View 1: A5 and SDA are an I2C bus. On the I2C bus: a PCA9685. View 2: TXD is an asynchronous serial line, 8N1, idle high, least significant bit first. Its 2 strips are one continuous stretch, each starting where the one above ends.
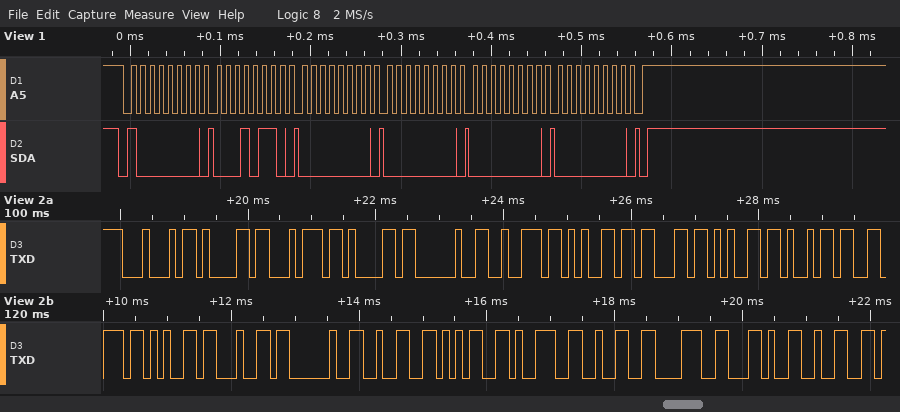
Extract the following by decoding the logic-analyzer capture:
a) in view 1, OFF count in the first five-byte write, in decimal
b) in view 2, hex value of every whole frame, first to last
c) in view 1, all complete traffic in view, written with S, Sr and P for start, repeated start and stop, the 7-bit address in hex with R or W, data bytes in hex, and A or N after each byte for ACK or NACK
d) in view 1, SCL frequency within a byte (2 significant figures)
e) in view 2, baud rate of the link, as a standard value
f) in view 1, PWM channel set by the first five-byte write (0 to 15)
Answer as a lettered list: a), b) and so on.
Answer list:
a) 0
b) 44 61 74 61 20 72 65 63 65 69 76 65 64 20 32 35 39 32 38 2C 32
c) S 40W A 16 A 00 A 00 A 00 A 00 A P
d) 100 kHz
e) 9600 baud
f) 4
